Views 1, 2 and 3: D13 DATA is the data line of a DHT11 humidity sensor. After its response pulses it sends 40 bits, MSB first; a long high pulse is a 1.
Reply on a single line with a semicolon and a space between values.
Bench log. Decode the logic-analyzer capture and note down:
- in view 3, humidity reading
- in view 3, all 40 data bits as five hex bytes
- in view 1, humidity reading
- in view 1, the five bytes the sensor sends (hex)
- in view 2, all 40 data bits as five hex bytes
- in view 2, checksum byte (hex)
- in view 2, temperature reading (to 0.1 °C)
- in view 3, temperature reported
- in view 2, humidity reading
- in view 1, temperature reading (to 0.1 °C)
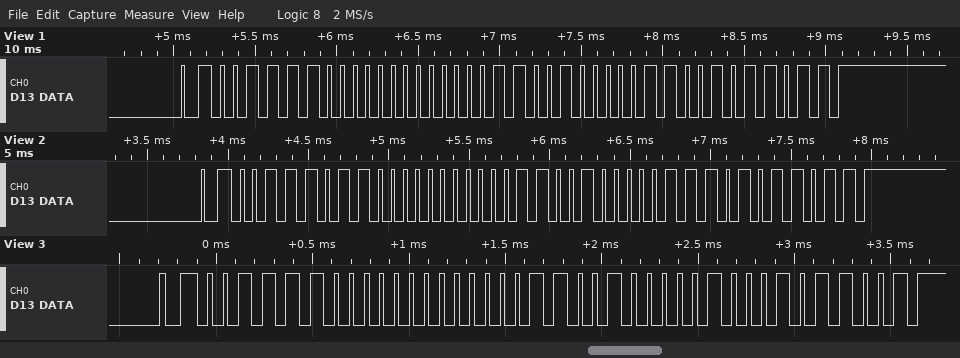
60 %; 3C 00 19 04 59; 60 %; 3C 00 19 06 5B; 3B 00 19 07 5B; 0x5B; 25.7 °C; 25.4 °C; 59 %; 25.6 °C
